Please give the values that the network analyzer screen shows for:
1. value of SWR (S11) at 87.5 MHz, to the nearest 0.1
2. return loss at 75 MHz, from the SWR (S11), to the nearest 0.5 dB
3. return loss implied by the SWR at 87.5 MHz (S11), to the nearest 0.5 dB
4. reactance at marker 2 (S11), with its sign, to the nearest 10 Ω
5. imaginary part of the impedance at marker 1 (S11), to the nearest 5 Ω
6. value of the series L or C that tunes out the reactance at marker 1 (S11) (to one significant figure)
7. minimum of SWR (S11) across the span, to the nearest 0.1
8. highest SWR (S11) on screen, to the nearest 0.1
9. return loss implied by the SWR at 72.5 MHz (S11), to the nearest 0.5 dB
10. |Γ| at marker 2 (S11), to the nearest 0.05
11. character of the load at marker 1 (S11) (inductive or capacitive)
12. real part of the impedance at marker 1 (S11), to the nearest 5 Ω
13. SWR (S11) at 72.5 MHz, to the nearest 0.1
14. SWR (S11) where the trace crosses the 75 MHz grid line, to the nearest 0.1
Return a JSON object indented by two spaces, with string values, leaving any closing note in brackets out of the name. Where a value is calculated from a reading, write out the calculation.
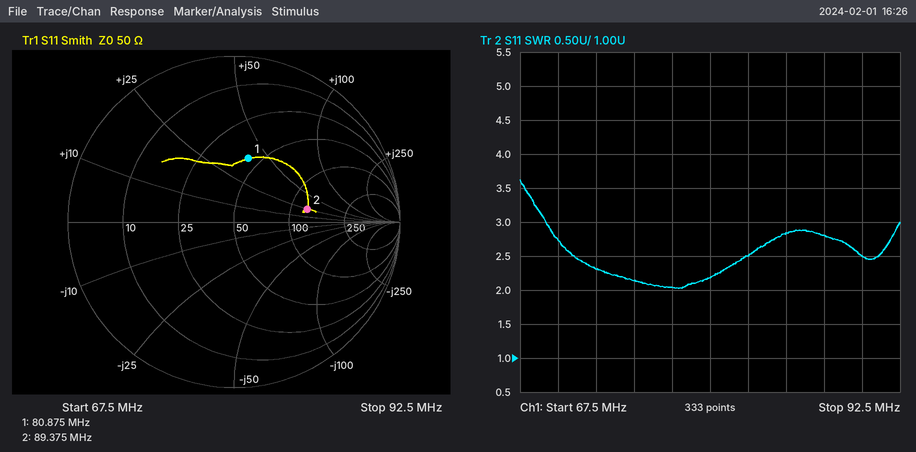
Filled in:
{
  "value of SWR (S11) at 87.5 MHz, to the nearest 0.1": "2.8",
  "return loss at 75 MHz, from the SWR (S11), to the nearest 0.5 dB": "−20 log10((2.1 − 1)/(2.1 + 1)) ≈ 9.0 dB",
  "return loss implied by the SWR at 87.5 MHz (S11), to the nearest 0.5 dB": "−20 log10((2.8 − 1)/(2.8 + 1)) ≈ 6.5 dB",
  "reactance at marker 2 (S11), with its sign, to the nearest 10 Ω": "+20 Ω",
  "imaginary part of the impedance at marker 1 (S11), to the nearest 5 Ω": "+40 Ω",
  "value of the series L or C that tunes out the reactance at marker 1 (S11)": "C = 1/(2π × 80.875 MHz × 40 Ω) ≈ 49.2 pF, so 50 pF to one significant figure",
  "minimum of SWR (S11) across the span, to the nearest 0.1": "2.0",
  "highest SWR (S11) on screen, to the nearest 0.1": "3.6",
  "return loss implied by the SWR at 72.5 MHz (S11), to the nearest 0.5 dB": "−20 log10((2.3 − 1)/(2.3 + 1)) ≈ 8.09 dB, so 8.0 dB to the nearest 0.5 dB",
  "|Γ| at marker 2 (S11), to the nearest 0.05": "0.45",
  "character of the load at marker 1 (S11)": "inductive",
  "real part of the impedance at marker 1 (S11), to the nearest 5 Ω": "45 Ω",
  "SWR (S11) at 72.5 MHz, to the nearest 0.1": "2.3",
  "SWR (S11) where the trace crosses the 75 MHz grid line, to the nearest 0.1": "2.1"
}
